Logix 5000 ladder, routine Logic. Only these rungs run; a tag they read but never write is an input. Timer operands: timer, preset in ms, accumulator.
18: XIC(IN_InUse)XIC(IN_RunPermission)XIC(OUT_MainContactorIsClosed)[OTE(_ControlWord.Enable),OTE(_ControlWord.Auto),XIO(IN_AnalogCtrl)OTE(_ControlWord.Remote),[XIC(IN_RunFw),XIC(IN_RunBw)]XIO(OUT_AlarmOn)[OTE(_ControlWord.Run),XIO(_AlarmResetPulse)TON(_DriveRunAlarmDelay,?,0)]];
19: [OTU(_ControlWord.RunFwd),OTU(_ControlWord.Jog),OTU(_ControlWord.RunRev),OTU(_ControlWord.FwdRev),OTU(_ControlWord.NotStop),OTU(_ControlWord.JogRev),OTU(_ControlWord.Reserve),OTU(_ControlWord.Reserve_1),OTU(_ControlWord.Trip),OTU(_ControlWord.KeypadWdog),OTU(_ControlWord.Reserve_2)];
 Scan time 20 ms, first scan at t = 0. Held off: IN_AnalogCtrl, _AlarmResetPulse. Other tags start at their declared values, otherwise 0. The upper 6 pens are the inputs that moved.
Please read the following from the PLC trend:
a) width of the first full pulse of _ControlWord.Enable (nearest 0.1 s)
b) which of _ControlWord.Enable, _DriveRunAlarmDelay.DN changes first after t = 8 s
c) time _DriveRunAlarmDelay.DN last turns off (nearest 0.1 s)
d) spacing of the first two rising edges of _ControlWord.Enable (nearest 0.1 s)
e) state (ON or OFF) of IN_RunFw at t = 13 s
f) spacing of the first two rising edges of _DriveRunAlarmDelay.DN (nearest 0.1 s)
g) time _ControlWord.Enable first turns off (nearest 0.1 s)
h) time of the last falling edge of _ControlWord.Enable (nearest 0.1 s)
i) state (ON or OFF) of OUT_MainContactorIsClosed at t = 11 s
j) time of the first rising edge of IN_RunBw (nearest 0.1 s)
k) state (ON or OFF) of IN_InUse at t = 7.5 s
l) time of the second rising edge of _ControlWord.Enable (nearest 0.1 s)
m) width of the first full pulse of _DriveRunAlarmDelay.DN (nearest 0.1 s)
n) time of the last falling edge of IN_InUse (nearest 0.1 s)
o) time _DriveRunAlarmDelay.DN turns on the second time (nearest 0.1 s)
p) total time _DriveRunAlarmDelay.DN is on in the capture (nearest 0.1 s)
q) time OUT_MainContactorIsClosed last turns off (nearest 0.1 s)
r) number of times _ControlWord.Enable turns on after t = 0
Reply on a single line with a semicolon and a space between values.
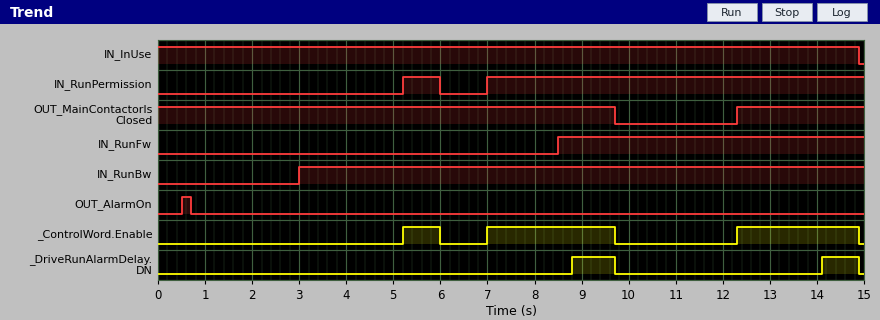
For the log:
0.8 s; _DriveRunAlarmDelay.DN; 14.9 s; 1.8 s; ON; 5.3 s; 6.0 s; 14.9 s; OFF; 3.0 s; ON; 7.0 s; 0.9 s; 14.9 s; 14.1 s; 1.7 s; 9.7 s; 3
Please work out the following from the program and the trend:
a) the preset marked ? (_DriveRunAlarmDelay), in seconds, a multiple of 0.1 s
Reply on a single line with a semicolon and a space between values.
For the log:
1.8 s
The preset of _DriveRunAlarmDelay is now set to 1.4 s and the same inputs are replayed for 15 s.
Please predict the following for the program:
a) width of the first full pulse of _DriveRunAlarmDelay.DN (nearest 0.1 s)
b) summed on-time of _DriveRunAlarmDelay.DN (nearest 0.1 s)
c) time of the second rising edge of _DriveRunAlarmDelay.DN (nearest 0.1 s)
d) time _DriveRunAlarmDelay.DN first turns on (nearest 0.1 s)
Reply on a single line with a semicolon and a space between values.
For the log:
1.3 s; 2.5 s; 13.7 s; 8.4 s
